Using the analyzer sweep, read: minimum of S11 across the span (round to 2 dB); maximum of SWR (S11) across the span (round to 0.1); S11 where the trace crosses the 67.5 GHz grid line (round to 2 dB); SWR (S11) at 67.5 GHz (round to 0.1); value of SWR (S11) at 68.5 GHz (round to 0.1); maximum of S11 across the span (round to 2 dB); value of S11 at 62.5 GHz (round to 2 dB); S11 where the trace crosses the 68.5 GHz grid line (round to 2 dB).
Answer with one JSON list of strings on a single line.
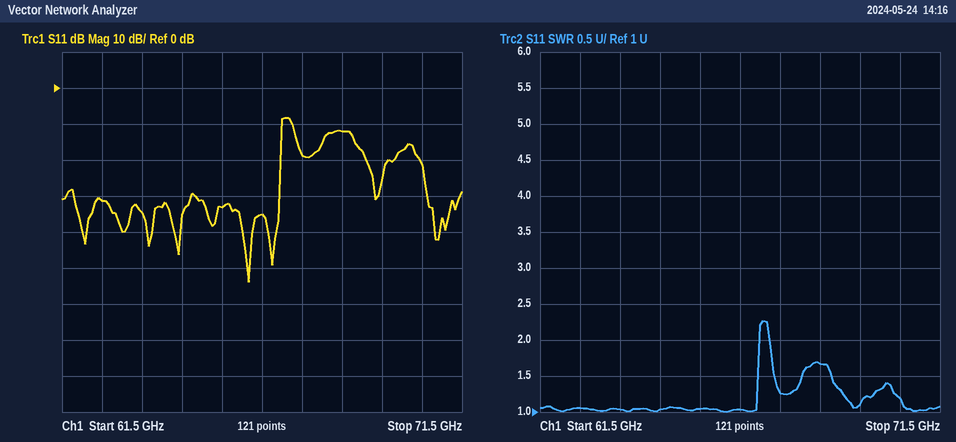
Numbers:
["-54 dB", "2.3", "-18 dB", "1.3", "1.7", "-8 dB", "-32 dB", "-12 dB"]
